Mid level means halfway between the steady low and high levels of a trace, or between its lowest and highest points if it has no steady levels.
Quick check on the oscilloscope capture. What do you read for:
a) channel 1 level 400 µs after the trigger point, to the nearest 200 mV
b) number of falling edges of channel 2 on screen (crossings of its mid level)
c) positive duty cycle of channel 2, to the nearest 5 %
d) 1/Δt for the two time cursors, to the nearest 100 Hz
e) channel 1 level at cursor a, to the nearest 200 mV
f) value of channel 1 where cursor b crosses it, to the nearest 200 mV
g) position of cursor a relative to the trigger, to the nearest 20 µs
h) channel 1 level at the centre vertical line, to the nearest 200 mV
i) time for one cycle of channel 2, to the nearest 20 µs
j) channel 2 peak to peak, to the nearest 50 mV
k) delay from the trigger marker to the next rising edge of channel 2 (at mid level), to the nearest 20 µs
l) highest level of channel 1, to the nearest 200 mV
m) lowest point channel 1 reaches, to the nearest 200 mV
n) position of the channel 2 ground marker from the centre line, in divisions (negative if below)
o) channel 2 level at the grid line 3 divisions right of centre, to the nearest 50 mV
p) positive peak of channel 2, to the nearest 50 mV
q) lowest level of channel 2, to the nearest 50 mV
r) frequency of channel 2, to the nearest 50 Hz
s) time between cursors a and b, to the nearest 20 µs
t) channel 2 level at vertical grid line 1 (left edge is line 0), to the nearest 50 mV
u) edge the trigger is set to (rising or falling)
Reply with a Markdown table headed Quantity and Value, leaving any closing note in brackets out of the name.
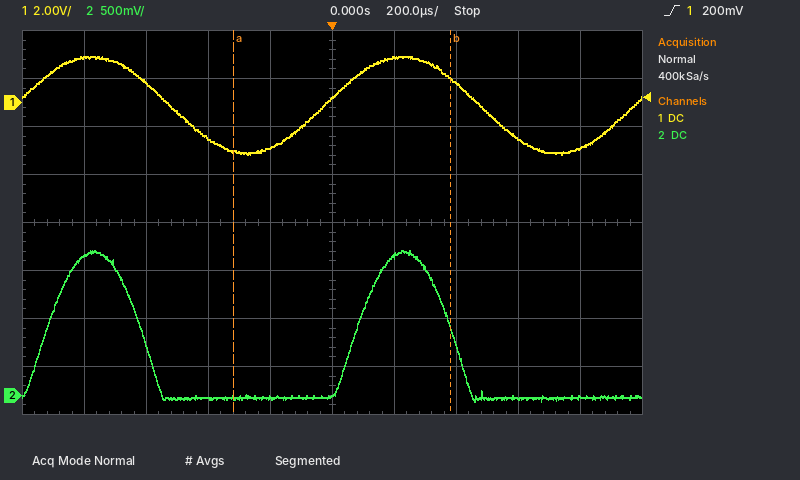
| Quantity | Value |
|---|---|
| channel 1 level 400 µs after the trigger point, to the nearest 200 mV | 800 mV |
| number of falling edges of channel 2 on screen | 2 |
| positive duty cycle of channel 2, to the nearest 5 % | 30 % |
| 1/Δt for the two time cursors, to the nearest 100 Hz | 1.4 kHz |
| channel 1 level at cursor a, to the nearest 200 mV | -2.0 V |
| value of channel 1 where cursor b crosses it, to the nearest 200 mV | 1.0 V |
| position of cursor a relative to the trigger, to the nearest 20 µs | -320 µs |
| channel 1 level at the centre vertical line, to the nearest 200 mV | 200 mV |
| time for one cycle of channel 2, to the nearest 20 µs | 1.00 ms |
| channel 2 peak to peak, to the nearest 50 mV | 1.55 V |
| delay from the trigger marker to the next rising edge of channel 2 (at mid level), to the nearest 20 µs | 80 µs |
| highest level of channel 1, to the nearest 200 mV | 2.0 V |
| lowest point channel 1 reaches, to the nearest 200 mV | -2.2 V |
| position of the channel 2 ground marker from the centre line, in divisions | -3.6 div |
| channel 2 level at the grid line 3 divisions right of centre, to the nearest 50 mV | -50 mV |
| positive peak of channel 2, to the nearest 50 mV | 1.50 V |
| lowest level of channel 2, to the nearest 50 mV | -50 mV |
| frequency of channel 2, to the nearest 50 Hz | 1.00 kHz |
| time between cursors a and b, to the nearest 20 µs | 700 µs |
| channel 2 level at vertical grid line 1 (left edge is line 0), to the nearest 50 mV | 1.45 V |
| edge the trigger is set to | rising |
